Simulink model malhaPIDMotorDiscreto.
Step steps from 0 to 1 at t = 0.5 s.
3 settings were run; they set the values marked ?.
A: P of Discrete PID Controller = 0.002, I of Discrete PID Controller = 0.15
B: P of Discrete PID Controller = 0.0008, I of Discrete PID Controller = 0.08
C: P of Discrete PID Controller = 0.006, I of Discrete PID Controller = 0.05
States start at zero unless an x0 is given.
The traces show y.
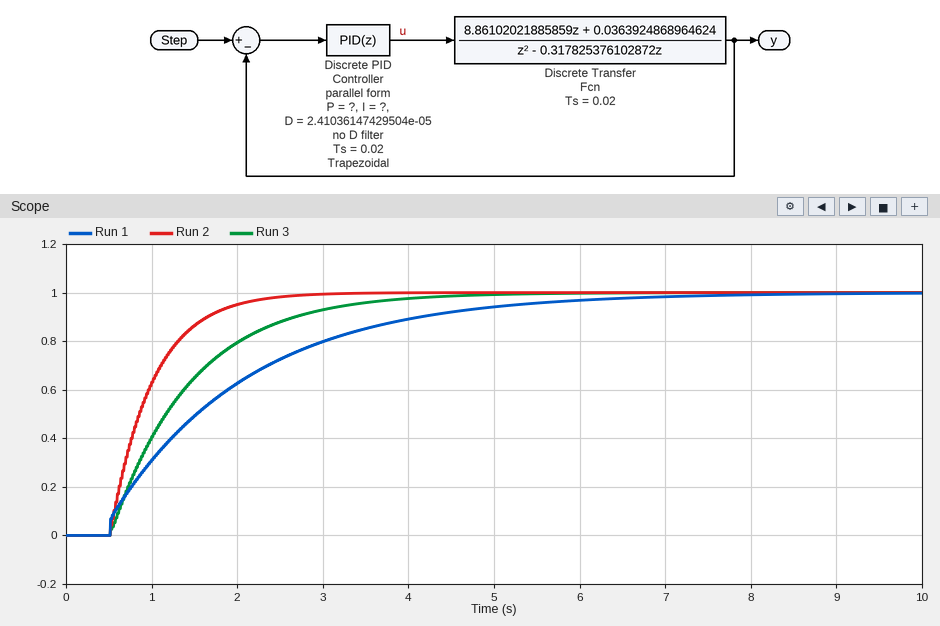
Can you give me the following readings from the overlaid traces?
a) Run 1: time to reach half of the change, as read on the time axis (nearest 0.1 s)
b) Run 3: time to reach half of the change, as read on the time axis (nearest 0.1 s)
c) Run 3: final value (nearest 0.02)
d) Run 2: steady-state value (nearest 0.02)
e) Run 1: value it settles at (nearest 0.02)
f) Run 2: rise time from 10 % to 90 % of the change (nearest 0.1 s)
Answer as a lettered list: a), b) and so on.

a) 1.5 s
b) 1.2 s
c) 1.00
d) 1.00
e) 1.00
f) 1.1 s
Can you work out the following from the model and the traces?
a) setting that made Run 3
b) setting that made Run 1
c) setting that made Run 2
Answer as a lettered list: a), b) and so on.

a) B
b) C
c) A
